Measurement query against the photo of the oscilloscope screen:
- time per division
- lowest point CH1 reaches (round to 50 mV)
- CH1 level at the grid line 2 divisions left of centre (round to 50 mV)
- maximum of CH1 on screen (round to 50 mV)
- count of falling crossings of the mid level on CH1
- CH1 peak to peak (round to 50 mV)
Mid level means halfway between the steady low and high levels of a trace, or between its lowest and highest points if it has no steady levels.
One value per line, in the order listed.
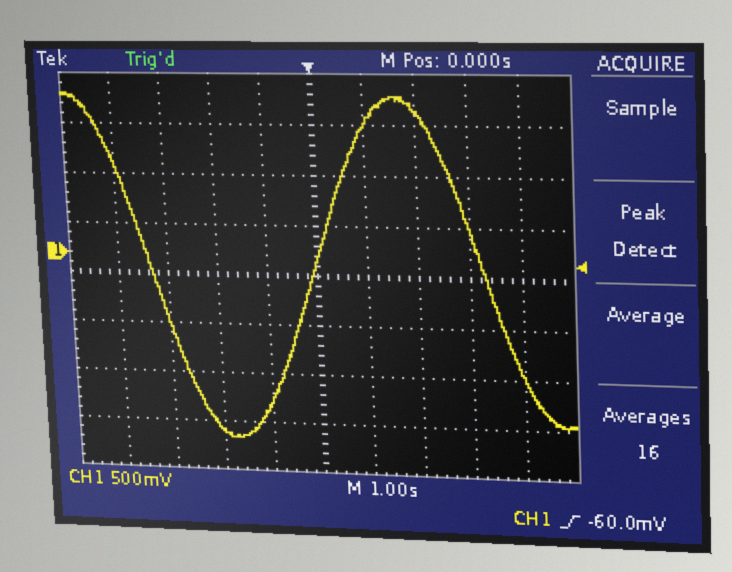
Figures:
1 s
-1.85 V
-1.80 V
1.60 V
2
3.45 V
